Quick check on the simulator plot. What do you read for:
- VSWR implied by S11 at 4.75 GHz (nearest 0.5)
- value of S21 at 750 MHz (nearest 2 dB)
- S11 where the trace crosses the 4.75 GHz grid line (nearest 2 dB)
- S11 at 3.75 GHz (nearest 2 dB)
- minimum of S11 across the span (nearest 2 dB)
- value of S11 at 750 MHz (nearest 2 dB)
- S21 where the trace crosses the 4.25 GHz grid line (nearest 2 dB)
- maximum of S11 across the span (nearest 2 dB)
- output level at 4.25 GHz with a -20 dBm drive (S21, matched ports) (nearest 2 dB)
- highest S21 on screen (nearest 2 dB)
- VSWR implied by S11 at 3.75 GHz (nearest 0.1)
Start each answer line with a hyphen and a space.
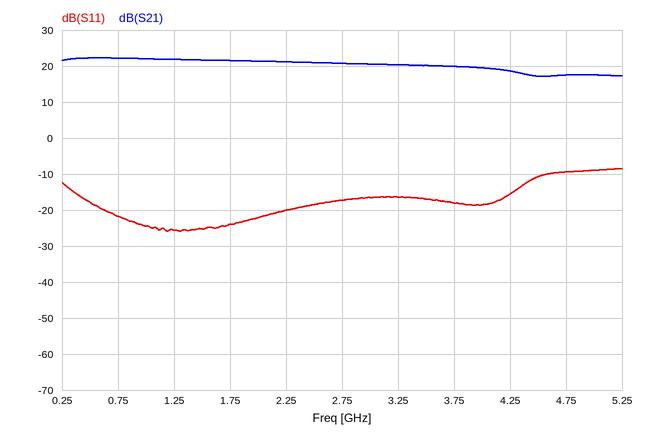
- 2.0
- 22 dB
- -10 dB
- -18 dB
- -26 dB
- -22 dB
- 18 dB
- -8 dB
- -2 dBm
- 22 dB
- 1.3
